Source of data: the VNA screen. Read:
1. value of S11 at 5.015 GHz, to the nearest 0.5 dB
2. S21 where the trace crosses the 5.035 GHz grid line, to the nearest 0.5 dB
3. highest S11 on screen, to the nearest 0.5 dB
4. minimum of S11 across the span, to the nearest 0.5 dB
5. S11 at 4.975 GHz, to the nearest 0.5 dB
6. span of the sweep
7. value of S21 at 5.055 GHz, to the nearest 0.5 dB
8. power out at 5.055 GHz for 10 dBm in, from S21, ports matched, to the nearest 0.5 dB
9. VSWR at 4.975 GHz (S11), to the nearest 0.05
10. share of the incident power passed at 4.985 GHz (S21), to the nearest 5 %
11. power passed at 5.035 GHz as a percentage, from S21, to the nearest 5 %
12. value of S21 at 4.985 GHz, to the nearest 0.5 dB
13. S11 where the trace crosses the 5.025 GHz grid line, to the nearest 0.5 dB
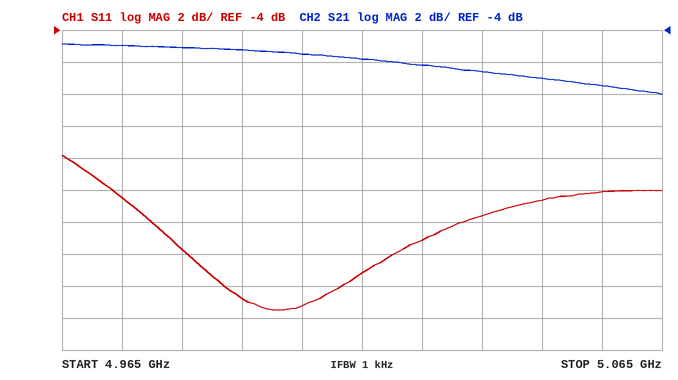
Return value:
-19.0 dB
-6.5 dB
-12.0 dB
-21.5 dB
-14.5 dB
100 MHz
-7.5 dB
2.5 dBm
1.45
30 %
20 %
-5.0 dB
-17.0 dB
